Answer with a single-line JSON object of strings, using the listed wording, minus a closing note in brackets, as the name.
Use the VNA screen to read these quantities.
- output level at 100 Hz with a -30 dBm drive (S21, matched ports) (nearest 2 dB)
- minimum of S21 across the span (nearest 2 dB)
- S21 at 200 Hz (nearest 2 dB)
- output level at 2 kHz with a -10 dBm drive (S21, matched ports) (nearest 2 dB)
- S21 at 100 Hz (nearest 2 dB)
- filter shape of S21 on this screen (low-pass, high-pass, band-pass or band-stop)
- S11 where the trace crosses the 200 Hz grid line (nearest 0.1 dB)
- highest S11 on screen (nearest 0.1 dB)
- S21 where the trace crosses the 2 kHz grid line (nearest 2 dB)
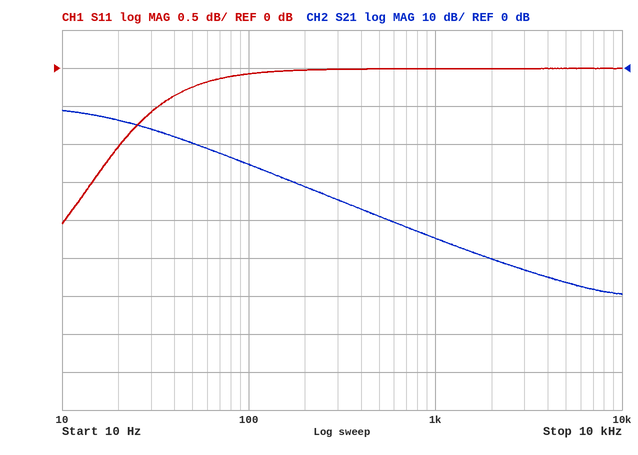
{"output level at 100 Hz with a -30 dBm drive (S21, matched ports)": "-56 dBm", "minimum of S21 across the span": "-60 dB", "S21 at 200 Hz": "-32 dB", "output level at 2 kHz with a -10 dBm drive (S21, matched ports)": "-60 dBm", "S21 at 100 Hz": "-26 dB", "filter shape of S21 on this screen": "low-pass", "S11 where the trace crosses the 200 Hz grid line": "0.0 dB", "highest S11 on screen": "0.0 dB", "S21 where the trace crosses the 2 kHz grid line": "-50 dB"}
